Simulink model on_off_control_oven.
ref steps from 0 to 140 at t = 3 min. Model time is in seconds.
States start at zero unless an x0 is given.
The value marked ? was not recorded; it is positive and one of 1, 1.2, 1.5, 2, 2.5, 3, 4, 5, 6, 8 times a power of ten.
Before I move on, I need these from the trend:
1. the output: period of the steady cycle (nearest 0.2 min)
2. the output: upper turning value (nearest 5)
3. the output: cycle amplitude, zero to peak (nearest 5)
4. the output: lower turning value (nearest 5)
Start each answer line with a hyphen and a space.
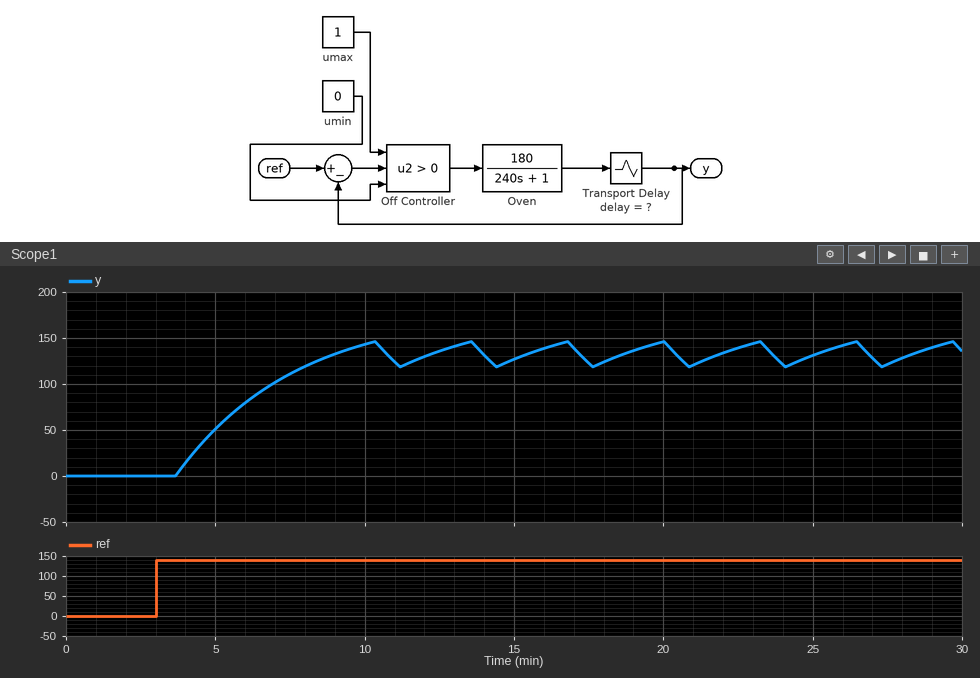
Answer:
- 3.2 min
- 145
- 15
- 120
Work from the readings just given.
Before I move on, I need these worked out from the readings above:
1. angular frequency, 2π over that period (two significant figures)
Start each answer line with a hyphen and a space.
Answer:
- 2.0 rad/min
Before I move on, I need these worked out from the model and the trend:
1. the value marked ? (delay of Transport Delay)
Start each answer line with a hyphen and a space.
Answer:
- 40
